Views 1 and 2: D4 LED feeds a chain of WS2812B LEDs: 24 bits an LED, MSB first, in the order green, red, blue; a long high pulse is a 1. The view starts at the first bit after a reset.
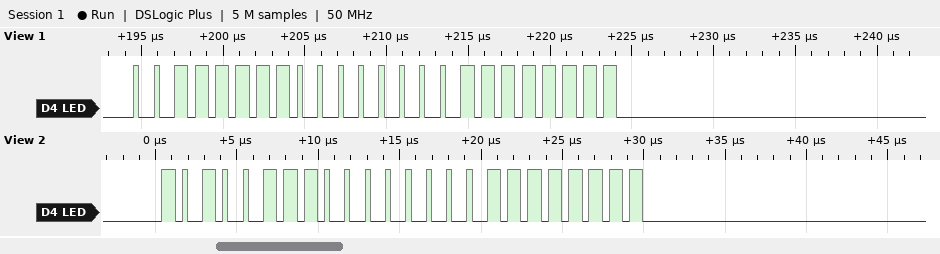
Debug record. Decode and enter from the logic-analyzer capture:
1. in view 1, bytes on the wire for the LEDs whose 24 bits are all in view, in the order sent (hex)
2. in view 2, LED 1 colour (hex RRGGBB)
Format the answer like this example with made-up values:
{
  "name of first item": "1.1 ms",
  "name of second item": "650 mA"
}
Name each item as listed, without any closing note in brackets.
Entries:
{
  "in view 1, bytes on the wire for the LEDs whose 24 bits are all in view, in the order sent": "3F 00 FF",
  "in view 2, LED 1 colour": "#00A7FF"
}
